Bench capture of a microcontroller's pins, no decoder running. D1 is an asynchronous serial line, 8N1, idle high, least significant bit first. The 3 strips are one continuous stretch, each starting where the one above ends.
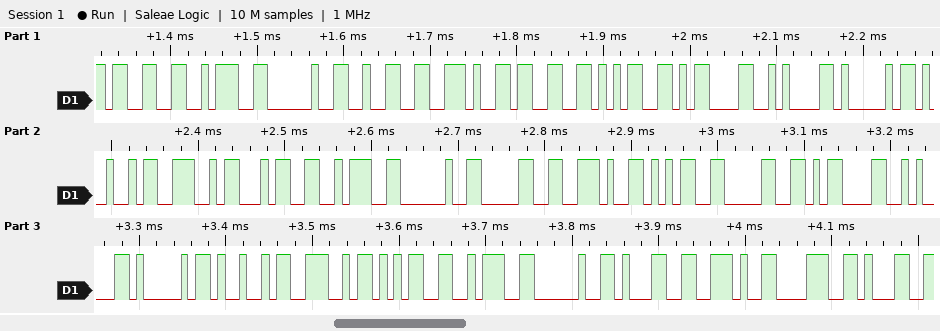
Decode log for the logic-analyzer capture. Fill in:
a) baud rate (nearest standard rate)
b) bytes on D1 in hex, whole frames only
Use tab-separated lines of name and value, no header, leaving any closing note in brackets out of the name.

baud rate	115200 baud
bytes on D1 in hex, whole frames only	33 3A 20 32 2E 33 35 0D 0A 41 49 4E 34 3A 20 30 2E 35 30 0D 0A 41 49 4E 35 3A 20 31 2E 38 31
